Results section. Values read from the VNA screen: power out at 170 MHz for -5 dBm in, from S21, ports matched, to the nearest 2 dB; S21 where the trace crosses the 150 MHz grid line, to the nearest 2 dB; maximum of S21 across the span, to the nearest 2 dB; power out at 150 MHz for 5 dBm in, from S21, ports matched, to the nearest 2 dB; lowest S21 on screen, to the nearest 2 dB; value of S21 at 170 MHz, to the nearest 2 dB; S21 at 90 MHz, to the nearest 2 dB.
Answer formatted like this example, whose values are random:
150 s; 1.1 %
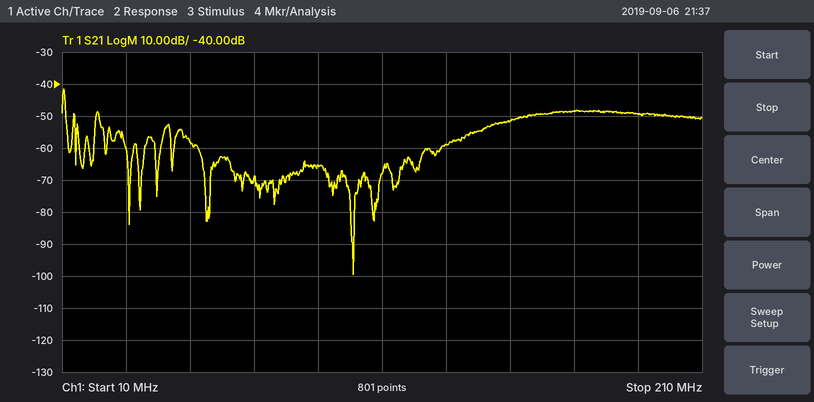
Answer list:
-54 dBm; -52 dB; -42 dB; -46 dBm; -100 dB; -48 dB; -66 dB
